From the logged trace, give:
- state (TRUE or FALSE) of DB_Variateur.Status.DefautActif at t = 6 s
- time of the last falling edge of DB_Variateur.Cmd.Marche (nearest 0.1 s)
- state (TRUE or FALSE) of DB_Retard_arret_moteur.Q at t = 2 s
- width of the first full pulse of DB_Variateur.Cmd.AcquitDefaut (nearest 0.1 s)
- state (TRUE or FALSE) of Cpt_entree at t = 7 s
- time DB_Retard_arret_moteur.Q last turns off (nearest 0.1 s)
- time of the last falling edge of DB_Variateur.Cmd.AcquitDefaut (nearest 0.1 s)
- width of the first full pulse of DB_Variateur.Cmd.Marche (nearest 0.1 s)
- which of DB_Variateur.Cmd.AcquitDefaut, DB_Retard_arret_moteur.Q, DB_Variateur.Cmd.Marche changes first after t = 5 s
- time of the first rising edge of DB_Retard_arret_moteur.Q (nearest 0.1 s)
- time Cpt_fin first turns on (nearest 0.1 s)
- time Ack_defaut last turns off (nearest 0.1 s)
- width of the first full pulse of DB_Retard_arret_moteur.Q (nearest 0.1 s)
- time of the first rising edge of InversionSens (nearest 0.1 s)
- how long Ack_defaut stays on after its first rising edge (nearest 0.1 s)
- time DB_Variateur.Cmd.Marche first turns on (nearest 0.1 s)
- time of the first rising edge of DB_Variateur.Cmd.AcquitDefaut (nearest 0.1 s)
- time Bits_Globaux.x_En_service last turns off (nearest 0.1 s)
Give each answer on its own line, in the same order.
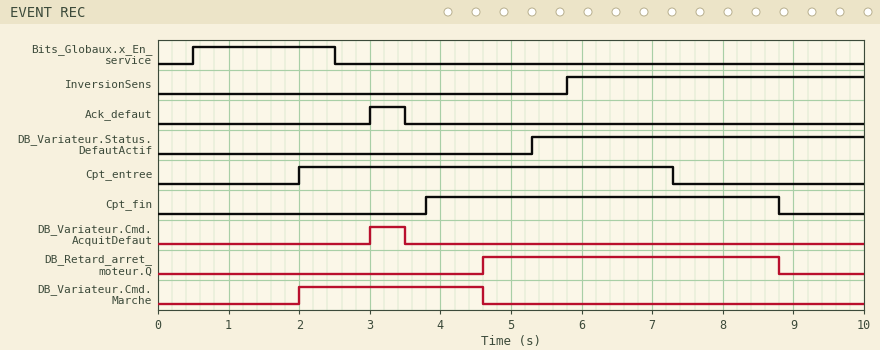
TRUE
4.6 s
FALSE
0.5 s
TRUE
8.8 s
3.5 s
2.6 s
DB_Retard_arret_moteur.Q
4.6 s
3.8 s
3.5 s
4.2 s
5.8 s
0.5 s
2.0 s
3.0 s
2.5 s
